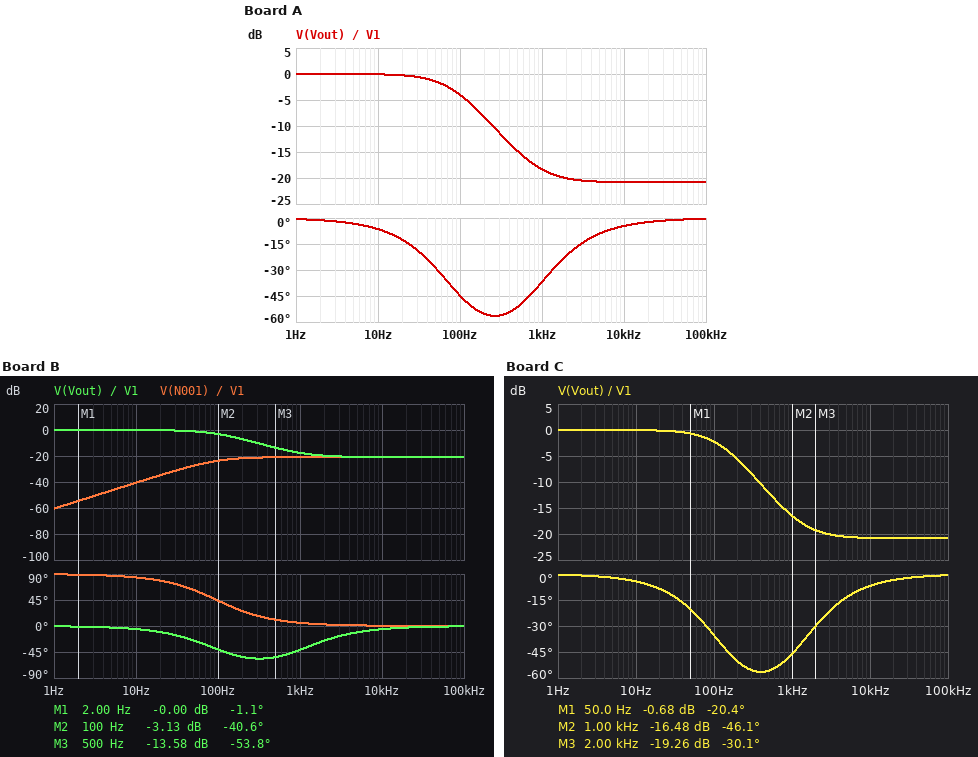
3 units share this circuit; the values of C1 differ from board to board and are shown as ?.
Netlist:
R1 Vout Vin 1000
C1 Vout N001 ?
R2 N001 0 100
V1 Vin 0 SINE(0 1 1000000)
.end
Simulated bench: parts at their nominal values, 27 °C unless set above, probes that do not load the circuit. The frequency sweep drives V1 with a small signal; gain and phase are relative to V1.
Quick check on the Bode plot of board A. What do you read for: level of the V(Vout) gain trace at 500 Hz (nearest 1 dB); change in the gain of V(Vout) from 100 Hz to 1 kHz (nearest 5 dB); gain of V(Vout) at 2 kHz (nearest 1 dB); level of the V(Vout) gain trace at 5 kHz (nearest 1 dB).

-15 dB
-15 dB
-20 dB
-21 dB
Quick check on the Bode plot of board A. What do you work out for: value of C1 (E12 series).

1.8 µF
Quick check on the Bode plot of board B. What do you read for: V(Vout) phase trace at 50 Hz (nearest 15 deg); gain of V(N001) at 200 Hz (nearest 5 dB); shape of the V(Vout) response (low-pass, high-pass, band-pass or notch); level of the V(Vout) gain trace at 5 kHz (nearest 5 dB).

-30 deg
-20 dB
low-pass
-20 dB
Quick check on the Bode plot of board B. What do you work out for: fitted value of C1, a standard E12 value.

1.5 µF
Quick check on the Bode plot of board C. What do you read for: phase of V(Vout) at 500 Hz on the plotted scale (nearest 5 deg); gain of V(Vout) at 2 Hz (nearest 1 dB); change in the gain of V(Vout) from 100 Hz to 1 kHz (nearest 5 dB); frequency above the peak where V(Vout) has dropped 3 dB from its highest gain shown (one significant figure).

-55 deg
0 dB
-15 dB
100 Hz
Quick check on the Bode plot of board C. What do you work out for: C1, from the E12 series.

1.2 µF
